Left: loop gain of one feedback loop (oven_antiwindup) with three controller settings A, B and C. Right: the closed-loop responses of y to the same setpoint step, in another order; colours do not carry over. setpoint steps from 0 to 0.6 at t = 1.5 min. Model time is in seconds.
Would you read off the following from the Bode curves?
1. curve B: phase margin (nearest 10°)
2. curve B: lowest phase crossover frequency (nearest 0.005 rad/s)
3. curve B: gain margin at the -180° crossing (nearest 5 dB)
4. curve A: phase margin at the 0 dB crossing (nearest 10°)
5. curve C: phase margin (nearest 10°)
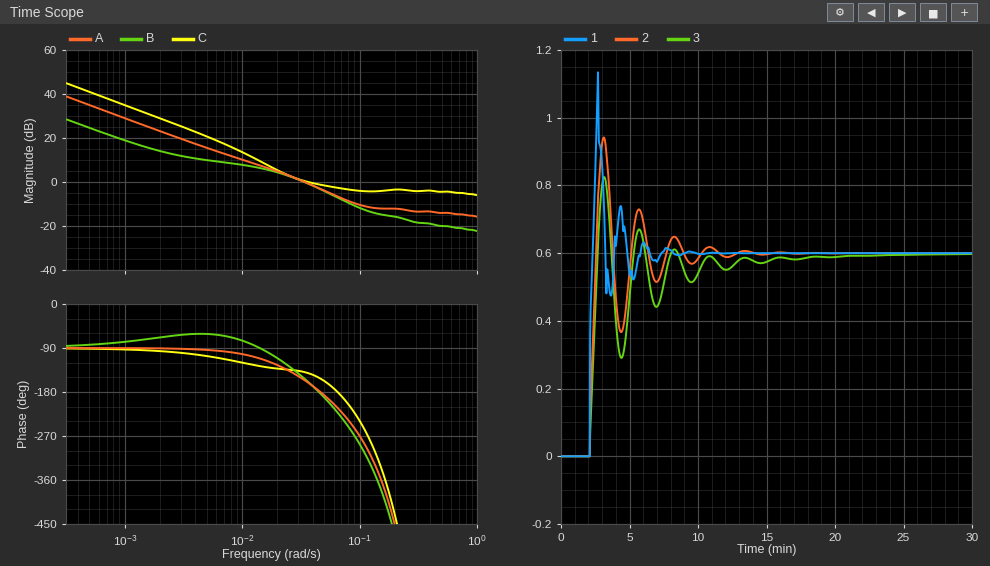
30°
0.045 rad/s
5 dB
20°
40°
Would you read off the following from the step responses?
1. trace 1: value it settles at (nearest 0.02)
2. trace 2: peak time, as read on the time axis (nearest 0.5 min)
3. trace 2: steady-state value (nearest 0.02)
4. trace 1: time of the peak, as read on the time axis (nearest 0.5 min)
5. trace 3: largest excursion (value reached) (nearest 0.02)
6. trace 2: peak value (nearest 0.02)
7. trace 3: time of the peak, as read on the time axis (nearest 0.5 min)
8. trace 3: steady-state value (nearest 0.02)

0.60
3.0 min
0.60
2.5 min
0.82
0.94
3.0 min
0.60
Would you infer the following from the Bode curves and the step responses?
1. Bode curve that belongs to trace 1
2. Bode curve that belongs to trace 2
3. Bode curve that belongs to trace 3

C
A
B
